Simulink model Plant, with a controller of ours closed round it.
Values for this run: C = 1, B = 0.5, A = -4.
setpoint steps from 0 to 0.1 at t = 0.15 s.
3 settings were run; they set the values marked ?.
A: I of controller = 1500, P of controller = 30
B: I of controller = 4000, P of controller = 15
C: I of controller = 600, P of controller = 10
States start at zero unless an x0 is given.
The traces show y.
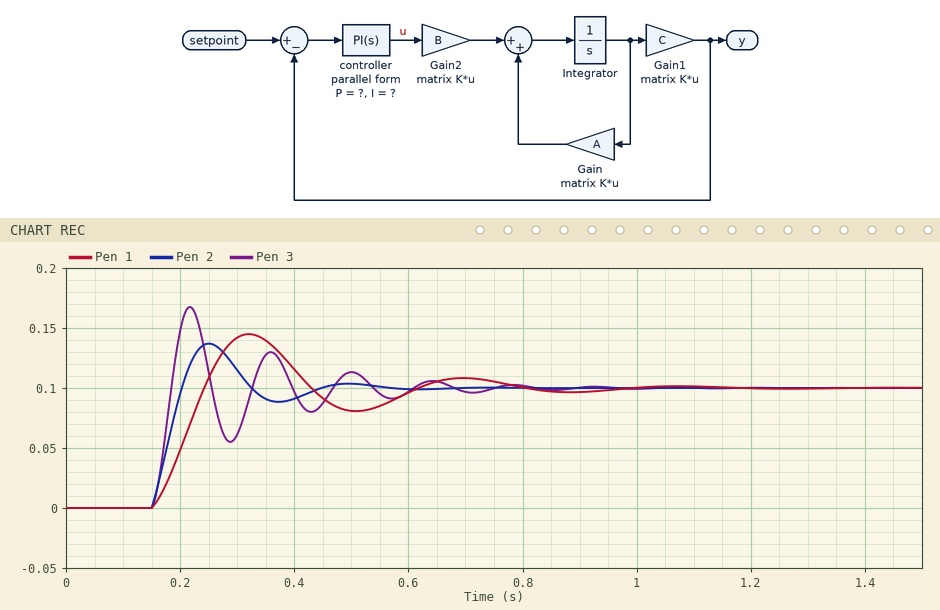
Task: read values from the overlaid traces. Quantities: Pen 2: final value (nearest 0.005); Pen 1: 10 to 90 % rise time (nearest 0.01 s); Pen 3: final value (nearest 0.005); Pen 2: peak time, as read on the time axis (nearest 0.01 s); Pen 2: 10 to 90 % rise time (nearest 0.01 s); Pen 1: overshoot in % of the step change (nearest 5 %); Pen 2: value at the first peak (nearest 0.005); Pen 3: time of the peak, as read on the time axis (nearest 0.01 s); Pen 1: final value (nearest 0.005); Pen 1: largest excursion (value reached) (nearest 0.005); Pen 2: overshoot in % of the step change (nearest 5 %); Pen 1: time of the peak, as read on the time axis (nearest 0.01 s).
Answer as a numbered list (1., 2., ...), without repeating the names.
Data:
1. 0.100
2. 0.07 s
3. 0.100
4. 0.25 s
5. 0.04 s
6. 45 %
7. 0.135
8. 0.22 s
9. 0.100
10. 0.145
11. 35 %
12. 0.32 s
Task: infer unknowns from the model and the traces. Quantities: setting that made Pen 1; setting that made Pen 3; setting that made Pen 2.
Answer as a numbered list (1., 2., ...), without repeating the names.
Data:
1. C
2. B
3. A
